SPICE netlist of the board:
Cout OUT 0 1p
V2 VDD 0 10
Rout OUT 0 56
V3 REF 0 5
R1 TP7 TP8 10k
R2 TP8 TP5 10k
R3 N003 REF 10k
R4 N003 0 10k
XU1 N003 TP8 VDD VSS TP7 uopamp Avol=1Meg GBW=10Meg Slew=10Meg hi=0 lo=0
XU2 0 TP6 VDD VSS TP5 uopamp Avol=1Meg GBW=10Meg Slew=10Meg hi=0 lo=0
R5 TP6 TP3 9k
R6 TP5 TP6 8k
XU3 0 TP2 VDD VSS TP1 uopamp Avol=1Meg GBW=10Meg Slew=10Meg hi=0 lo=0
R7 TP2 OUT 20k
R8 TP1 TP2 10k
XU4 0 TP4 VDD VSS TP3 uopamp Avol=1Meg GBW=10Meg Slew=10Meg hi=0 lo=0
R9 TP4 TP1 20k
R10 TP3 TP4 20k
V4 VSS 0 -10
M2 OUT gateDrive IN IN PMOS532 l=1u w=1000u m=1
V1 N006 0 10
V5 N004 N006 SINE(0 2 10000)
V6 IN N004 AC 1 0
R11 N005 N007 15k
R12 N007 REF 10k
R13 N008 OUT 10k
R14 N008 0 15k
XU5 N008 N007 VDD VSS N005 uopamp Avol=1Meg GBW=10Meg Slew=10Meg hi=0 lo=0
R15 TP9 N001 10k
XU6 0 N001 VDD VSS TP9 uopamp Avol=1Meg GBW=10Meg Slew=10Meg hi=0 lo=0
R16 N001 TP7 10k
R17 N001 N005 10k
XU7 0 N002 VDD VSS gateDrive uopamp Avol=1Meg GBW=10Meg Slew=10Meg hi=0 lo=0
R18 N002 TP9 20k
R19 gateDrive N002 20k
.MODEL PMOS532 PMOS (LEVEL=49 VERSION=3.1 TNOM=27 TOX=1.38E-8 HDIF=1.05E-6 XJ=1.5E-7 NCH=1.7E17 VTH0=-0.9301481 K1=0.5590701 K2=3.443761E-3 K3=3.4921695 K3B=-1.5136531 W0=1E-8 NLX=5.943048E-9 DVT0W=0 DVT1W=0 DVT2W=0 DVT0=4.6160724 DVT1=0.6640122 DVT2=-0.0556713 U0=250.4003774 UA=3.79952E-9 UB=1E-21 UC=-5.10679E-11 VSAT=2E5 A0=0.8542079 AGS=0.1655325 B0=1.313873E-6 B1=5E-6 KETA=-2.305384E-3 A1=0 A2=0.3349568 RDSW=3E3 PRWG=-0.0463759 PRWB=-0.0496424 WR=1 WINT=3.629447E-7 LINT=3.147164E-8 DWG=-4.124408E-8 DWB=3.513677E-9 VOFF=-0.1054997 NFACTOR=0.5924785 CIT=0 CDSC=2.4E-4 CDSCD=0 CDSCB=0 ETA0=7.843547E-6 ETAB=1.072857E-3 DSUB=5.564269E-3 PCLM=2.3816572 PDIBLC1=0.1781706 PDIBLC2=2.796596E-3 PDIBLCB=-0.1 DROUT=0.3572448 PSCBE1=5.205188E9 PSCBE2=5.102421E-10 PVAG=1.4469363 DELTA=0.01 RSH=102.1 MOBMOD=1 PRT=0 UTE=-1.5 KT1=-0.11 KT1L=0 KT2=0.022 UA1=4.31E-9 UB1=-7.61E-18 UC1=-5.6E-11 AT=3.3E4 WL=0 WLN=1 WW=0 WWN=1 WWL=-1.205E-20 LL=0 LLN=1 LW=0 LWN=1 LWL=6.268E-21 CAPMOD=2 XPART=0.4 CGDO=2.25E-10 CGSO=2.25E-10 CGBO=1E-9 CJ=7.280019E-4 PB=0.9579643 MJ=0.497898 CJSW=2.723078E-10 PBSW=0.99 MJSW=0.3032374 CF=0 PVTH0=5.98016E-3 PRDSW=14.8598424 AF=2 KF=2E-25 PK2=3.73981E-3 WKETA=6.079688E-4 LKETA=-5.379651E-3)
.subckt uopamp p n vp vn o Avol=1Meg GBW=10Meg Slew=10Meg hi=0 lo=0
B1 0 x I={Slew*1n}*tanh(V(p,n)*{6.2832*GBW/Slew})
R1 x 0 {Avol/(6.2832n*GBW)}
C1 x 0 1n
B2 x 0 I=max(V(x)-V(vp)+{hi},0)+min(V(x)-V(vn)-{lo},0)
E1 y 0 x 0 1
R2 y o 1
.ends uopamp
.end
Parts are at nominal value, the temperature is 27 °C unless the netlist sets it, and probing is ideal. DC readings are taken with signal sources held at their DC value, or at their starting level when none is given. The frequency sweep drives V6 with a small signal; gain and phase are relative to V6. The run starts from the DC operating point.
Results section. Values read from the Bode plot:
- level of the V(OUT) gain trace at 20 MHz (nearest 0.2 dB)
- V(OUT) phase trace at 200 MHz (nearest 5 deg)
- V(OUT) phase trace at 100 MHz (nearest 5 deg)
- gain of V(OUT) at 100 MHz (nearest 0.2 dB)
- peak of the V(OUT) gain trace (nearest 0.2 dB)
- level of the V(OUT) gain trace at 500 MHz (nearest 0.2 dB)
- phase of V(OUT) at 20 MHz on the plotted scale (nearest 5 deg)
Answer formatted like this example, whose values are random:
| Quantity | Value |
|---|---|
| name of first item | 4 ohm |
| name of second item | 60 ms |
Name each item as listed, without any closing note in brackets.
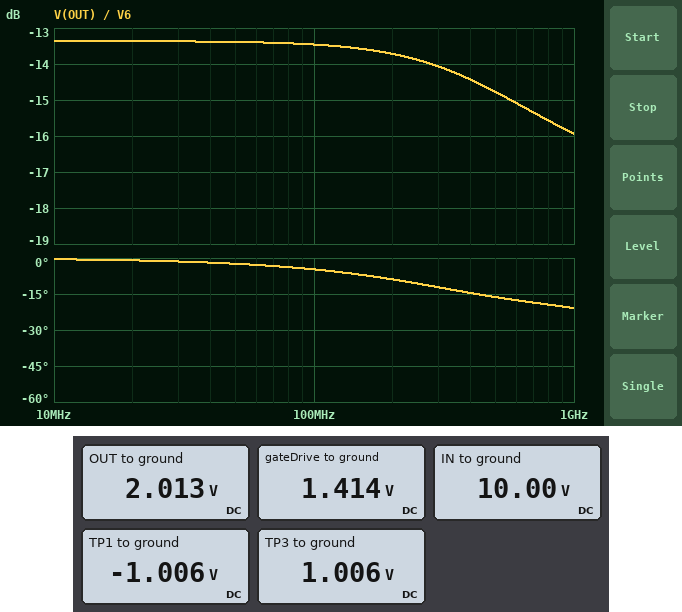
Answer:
| Quantity | Value |
|---|---|
| level of the V(OUT) gain trace at 20 MHz | -13.4 dB |
| V(OUT) phase trace at 200 MHz | -10 deg |
| V(OUT) phase trace at 100 MHz | -5 deg |
| gain of V(OUT) at 100 MHz | -13.4 dB |
| peak of the V(OUT) gain trace | -13.4 dB |
| level of the V(OUT) gain trace at 500 MHz | -14.8 dB |
| phase of V(OUT) at 20 MHz on the plotted scale | 0 deg |
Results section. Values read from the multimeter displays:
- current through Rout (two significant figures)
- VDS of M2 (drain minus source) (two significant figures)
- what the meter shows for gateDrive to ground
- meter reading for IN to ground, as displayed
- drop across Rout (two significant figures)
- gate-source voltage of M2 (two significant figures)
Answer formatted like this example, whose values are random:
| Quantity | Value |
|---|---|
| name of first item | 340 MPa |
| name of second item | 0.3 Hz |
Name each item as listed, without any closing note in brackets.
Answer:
| Quantity | Value |
|---|---|
| current through Rout | 36 mA |
| VDS of M2 (drain minus source) | -8.0 V |
| what the meter shows for gateDrive to ground | 1.414 V |
| meter reading for IN to ground, as displayed | 10.00 V |
| drop across Rout | 2.0 V |
| gate-source voltage of M2 | -8.6 V |
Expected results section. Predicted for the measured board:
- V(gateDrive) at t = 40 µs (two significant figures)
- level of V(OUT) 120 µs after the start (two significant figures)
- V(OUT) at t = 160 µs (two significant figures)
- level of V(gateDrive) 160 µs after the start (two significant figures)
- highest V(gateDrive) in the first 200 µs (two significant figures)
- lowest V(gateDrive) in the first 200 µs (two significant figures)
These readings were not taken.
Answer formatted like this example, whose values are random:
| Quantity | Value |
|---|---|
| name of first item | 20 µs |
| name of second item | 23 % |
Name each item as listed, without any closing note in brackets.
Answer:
| Quantity | Value |
|---|---|
| V(gateDrive) at t = 40 µs | 1.9 V |
| level of V(OUT) 120 µs after the start | 2.4 V |
| V(OUT) at t = 160 µs | 1.8 V |
| level of V(gateDrive) 160 µs after the start | 950 mV |
| highest V(gateDrive) in the first 200 µs | 2.2 V |
| lowest V(gateDrive) in the first 200 µs | 620 mV |
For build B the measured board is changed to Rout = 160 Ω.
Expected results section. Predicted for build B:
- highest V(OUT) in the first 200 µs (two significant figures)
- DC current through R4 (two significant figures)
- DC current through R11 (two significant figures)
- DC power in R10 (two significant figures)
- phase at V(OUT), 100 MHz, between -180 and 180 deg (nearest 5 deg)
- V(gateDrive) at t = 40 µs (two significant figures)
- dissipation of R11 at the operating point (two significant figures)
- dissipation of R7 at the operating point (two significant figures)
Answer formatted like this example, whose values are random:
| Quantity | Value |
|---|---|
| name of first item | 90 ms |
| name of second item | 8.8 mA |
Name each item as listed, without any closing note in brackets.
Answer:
| Quantity | Value |
|---|---|
| highest V(OUT) in the first 200 µs | 4.5 V |
| DC current through R4 | 250 µA |
| DC current through R11 | 270 µA |
| DC power in R10 | 180 µW |
| phase at V(OUT), 100 MHz, between -180 and 180 deg | -10 deg |
| V(gateDrive) at t = 40 µs | 5.6 V |
| dissipation of R11 at the operating point | 1.1 mW |
| dissipation of R7 at the operating point | 710 µW |
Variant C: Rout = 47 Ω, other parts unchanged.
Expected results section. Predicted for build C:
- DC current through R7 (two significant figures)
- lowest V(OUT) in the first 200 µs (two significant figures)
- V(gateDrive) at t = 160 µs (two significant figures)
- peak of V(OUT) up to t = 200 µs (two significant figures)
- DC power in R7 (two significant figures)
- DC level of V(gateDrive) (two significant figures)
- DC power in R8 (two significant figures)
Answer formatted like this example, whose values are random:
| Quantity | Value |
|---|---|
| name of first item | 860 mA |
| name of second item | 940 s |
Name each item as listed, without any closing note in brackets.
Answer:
| Quantity | Value |
|---|---|
| DC current through R7 | 88 µA |
| lowest V(OUT) in the first 200 µs | 1.4 V |
| V(gateDrive) at t = 160 µs | 510 mV |
| peak of V(OUT) up to t = 200 µs | 2.1 V |
| DC power in R7 | 150 µW |
| DC level of V(gateDrive) | 910 mV |
| DC power in R8 | 77 µW |
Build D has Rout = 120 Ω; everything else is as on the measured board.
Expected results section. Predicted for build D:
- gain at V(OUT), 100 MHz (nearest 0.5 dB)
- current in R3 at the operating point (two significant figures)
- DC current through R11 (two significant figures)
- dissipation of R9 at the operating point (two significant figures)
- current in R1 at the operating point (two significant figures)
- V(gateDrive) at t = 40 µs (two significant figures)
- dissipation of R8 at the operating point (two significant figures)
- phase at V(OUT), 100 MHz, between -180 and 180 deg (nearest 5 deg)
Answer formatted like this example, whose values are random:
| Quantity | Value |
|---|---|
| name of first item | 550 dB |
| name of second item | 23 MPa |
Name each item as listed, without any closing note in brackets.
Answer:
| Quantity | Value |
|---|---|
| gain at V(OUT), 100 MHz | -6.5 dB |
| current in R3 at the operating point | 250 µA |
| DC current through R11 | 300 µA |
| dissipation of R9 at the operating point | 140 µW |
| current in R1 at the operating point | 400 µA |
| V(gateDrive) at t = 40 µs | 4.7 V |
| dissipation of R8 at the operating point | 280 µW |
| phase at V(OUT), 100 MHz, between -180 and 180 deg | -10 deg |
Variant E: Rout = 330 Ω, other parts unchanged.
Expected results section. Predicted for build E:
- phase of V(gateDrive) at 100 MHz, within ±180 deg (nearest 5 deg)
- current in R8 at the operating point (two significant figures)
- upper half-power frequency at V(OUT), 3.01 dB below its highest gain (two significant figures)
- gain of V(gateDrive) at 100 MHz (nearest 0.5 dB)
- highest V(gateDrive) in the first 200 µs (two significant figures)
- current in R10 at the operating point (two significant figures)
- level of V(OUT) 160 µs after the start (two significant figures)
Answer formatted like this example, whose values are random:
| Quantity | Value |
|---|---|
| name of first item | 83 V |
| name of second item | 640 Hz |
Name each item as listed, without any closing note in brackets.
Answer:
| Quantity | Value |
|---|---|
| phase of V(gateDrive) at 100 MHz, within ±180 deg | 85 deg |
| current in R8 at the operating point | 230 µA |
| upper half-power frequency at V(OUT), 3.01 dB below its highest gain | 6.4 MHz |
| gain of V(gateDrive) at 100 MHz | -60.0 dB |
| highest V(gateDrive) in the first 200 µs | 8.0 V |
| current in R10 at the operating point | 110 µA |
| level of V(OUT) 160 µs after the start | 4.1 V |
